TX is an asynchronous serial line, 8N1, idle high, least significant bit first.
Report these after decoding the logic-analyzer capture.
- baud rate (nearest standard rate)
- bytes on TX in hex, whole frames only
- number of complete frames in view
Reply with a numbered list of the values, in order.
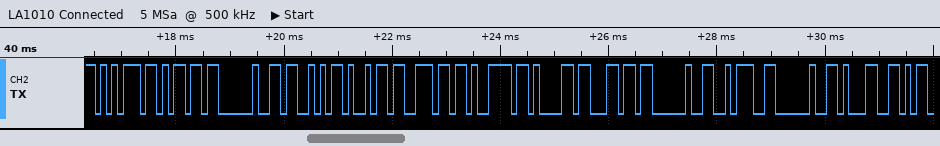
1. 9600 baud
2. 0x75 0x6D 0x20 0x53 0x69 0x6E 0x79 0x61 0x6C 0x20 0x3A 0x20 0x31
3. 13
